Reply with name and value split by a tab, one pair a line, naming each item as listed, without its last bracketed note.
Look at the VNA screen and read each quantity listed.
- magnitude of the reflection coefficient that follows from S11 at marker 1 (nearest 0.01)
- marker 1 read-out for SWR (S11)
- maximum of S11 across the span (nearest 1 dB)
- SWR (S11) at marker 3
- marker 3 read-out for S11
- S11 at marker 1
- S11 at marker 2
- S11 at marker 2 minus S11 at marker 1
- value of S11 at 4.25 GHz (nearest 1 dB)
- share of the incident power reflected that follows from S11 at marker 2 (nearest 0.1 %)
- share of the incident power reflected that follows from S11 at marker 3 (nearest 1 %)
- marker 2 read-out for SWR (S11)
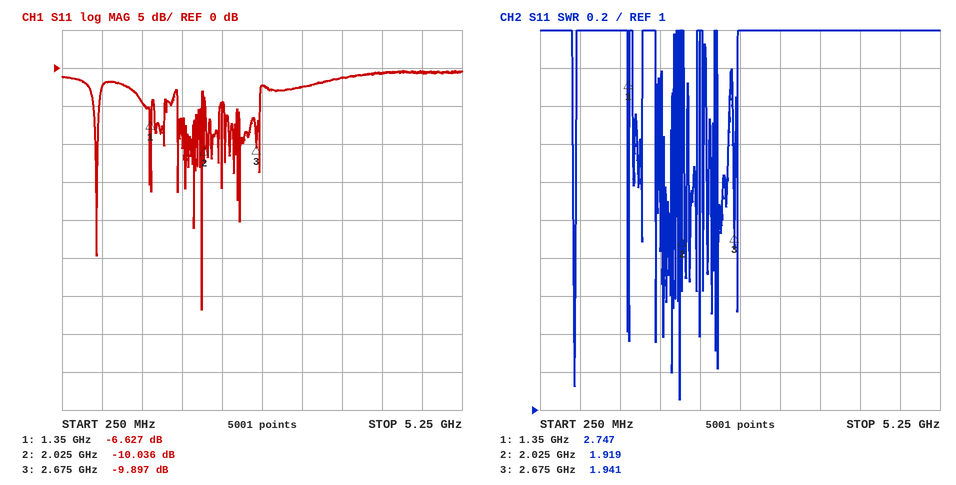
magnitude of the reflection coefficient that follows from S11 at marker 1	0.47
marker 1 read-out for SWR	2.747
maximum of S11 across the span	0 dB
SWR (S11) at marker 3	1.941
marker 3 read-out for S11	-9.897 dB
S11 at marker 1	-6.627 dB
S11 at marker 2	-10.036 dB
S11 at marker 2 minus S11 at marker 1	-3.409 dB
value of S11 at 4.25 GHz	-1 dB
share of the incident power reflected that follows from S11 at marker 2	9.9 %
share of the incident power reflected that follows from S11 at marker 3	10 %
marker 2 read-out for SWR	1.919
